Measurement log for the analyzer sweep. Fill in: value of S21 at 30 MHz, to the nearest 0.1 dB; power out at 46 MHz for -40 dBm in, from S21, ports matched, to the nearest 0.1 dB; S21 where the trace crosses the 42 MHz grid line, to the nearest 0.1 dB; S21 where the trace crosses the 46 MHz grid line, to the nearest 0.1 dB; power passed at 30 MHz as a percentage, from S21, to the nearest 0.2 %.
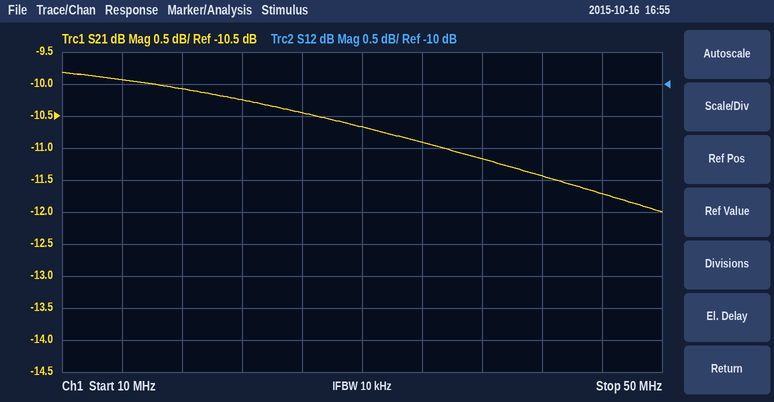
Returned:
-10.7 dB
-51.7 dBm
-11.4 dB
-11.7 dB
8.6 %
